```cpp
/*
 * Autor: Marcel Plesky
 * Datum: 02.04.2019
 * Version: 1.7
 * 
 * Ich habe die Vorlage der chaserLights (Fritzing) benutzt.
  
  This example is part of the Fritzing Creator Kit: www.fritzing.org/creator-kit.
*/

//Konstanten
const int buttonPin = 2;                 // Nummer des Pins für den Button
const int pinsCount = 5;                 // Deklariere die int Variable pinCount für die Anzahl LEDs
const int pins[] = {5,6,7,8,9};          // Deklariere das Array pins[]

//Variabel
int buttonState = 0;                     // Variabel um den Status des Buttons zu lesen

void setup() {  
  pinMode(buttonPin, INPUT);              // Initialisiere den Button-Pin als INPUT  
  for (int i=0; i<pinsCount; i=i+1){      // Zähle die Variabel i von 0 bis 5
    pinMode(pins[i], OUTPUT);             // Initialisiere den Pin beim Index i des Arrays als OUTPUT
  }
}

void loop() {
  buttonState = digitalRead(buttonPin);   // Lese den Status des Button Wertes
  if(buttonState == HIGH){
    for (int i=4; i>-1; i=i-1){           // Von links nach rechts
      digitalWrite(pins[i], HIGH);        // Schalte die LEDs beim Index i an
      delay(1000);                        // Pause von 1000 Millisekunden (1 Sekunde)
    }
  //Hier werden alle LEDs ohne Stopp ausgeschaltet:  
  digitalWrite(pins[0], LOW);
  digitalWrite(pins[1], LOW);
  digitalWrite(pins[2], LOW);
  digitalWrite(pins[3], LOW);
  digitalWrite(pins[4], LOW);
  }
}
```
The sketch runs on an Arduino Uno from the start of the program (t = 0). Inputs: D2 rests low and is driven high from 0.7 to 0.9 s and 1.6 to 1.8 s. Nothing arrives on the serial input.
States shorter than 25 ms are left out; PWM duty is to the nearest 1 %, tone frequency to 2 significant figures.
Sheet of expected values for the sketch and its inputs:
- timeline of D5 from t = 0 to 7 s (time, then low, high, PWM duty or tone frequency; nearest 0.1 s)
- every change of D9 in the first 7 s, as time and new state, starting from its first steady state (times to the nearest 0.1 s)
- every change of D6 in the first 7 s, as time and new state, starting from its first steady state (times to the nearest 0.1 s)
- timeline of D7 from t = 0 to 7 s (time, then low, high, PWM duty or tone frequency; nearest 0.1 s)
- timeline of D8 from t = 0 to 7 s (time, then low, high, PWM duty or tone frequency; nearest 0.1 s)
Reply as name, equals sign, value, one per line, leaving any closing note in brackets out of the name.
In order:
timeline of D5 from t = 0 to 7 s = 0 s low; 4.7 s high; 5.7 s low
every change of D9 in the first 7 s, as time and new state, starting from its first steady state = 0 s low; 0.7 s high; 5.7 s low
every change of D6 in the first 7 s, as time and new state, starting from its first steady state = 0 s low; 3.7 s high; 5.7 s low
timeline of D7 from t = 0 to 7 s = 0 s low; 2.7 s high; 5.7 s low
timeline of D8 from t = 0 to 7 s = 0 s low; 1.7 s high; 5.7 s low
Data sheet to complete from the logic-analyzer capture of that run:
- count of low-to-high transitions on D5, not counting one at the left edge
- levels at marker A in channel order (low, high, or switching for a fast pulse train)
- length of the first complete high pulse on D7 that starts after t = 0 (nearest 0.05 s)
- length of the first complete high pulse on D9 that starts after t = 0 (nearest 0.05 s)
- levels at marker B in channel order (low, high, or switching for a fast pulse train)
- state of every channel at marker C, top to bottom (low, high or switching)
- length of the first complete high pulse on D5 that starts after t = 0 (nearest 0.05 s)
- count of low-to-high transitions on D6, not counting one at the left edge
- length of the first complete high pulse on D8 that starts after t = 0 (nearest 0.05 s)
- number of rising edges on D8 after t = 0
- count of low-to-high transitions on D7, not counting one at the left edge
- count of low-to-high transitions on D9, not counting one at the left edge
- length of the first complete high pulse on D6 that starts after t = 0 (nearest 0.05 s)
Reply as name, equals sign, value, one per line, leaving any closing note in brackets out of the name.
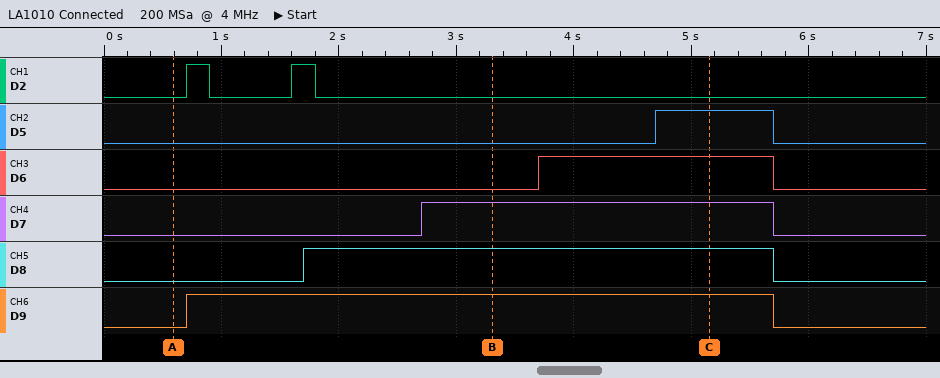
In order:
count of low-to-high transitions on D5, not counting one at the left edge = 1
levels at marker A in channel order = D2 low, D5 low, D6 low, D7 low, D8 low, D9 low
length of the first complete high pulse on D7 that starts after t = 0 = 3.00 s
length of the first complete high pulse on D9 that starts after t = 0 = 5.00 s
levels at marker B in channel order = D2 low, D5 low, D6 low, D7 high, D8 high, D9 high
state of every channel at marker C, top to bottom = D2 low, D5 high, D6 high, D7 high, D8 high, D9 high
length of the first complete high pulse on D5 that starts after t = 0 = 1.00 s
count of low-to-high transitions on D6, not counting one at the left edge = 1
length of the first complete high pulse on D8 that starts after t = 0 = 4.00 s
number of rising edges on D8 after t = 0 = 1
count of low-to-high transitions on D7, not counting one at the left edge = 1
count of low-to-high transitions on D9, not counting one at the left edge = 1
length of the first complete high pulse on D6 that starts after t = 0 = 2.00 s
